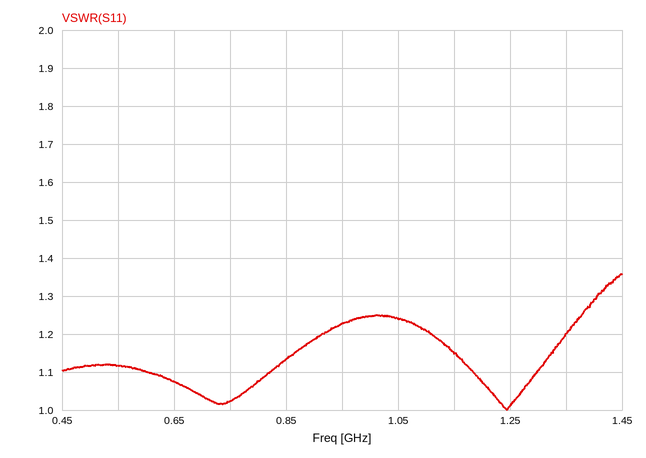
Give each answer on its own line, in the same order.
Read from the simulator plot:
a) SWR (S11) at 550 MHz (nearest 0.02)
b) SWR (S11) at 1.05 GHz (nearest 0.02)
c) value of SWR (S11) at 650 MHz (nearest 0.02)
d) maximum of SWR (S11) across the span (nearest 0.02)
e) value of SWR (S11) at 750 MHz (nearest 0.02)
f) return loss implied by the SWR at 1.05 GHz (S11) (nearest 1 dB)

1.12
1.24
1.08
1.36
1.02
19 dB
